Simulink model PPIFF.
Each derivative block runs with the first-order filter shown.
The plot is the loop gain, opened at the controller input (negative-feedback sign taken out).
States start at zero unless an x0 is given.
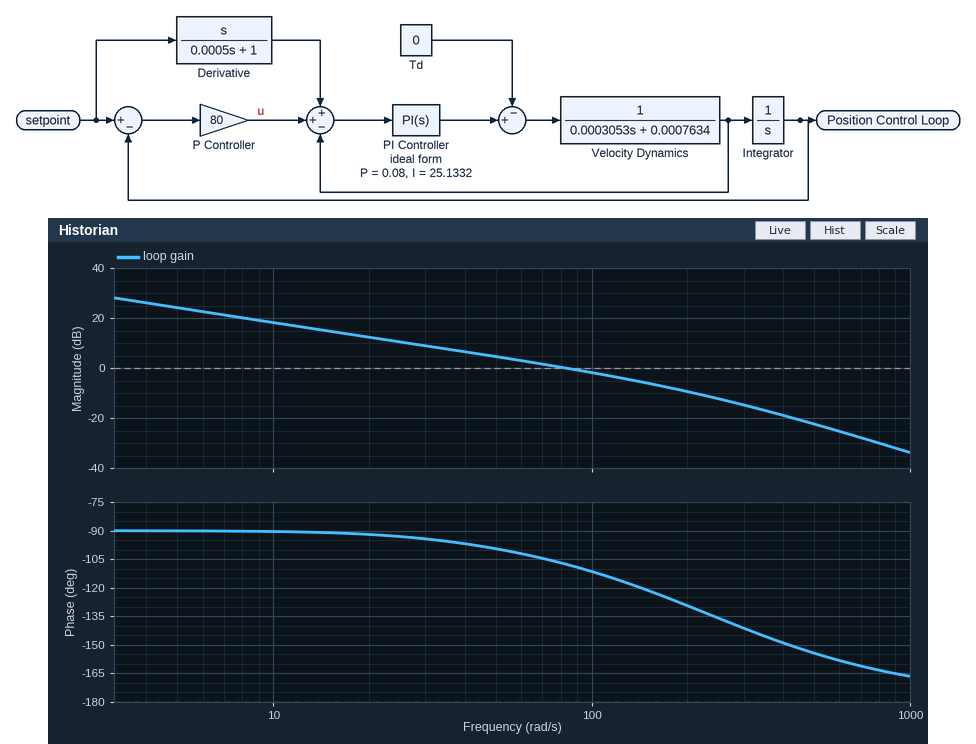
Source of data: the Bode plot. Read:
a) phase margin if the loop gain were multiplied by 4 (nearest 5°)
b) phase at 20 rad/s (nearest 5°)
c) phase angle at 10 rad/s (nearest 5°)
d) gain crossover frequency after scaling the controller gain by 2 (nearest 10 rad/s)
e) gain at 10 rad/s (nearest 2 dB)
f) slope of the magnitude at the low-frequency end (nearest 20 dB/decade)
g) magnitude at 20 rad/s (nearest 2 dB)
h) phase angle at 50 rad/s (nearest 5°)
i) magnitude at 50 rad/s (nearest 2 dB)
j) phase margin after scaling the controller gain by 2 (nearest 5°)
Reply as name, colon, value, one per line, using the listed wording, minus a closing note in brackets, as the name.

phase margin if the loop gain were multiplied by 4: 45°
phase at 20 rad/s: -90°
phase angle at 10 rad/s: -90°
gain crossover frequency after scaling the controller gain by 2: 150 rad/s
gain at 10 rad/s: 18 dB
slope of the magnitude at the low-frequency end: -20 dB/decade
magnitude at 20 rad/s: 12 dB
phase angle at 50 rad/s: -100°
magnitude at 50 rad/s: 4 dB
phase margin after scaling the controller gain by 2: 60°
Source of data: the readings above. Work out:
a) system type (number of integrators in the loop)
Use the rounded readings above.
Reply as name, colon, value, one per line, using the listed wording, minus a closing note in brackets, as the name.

system type: 1
